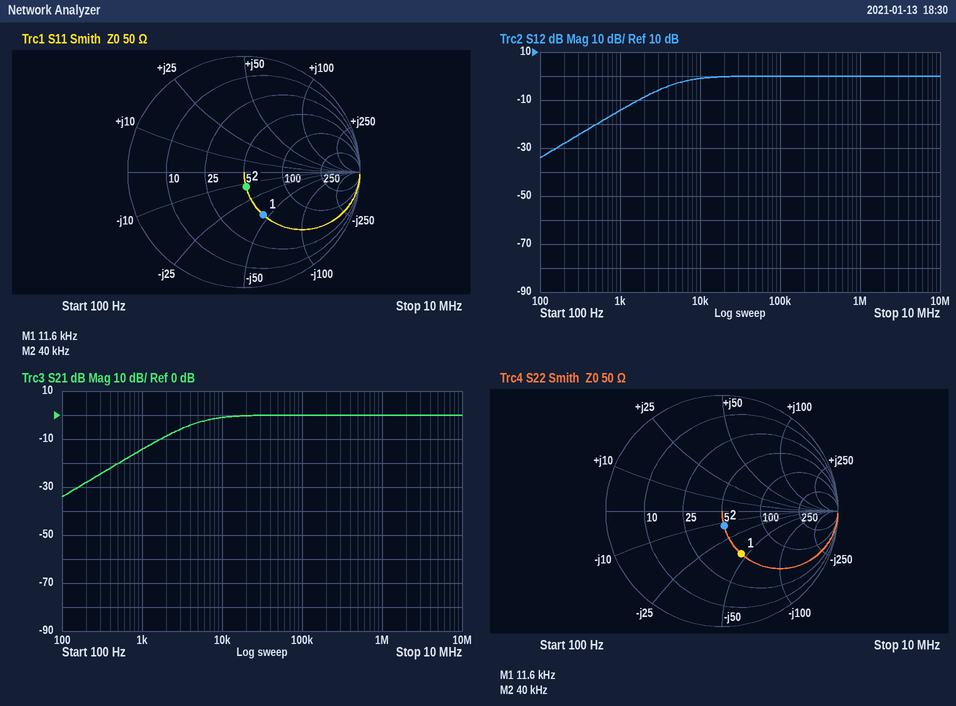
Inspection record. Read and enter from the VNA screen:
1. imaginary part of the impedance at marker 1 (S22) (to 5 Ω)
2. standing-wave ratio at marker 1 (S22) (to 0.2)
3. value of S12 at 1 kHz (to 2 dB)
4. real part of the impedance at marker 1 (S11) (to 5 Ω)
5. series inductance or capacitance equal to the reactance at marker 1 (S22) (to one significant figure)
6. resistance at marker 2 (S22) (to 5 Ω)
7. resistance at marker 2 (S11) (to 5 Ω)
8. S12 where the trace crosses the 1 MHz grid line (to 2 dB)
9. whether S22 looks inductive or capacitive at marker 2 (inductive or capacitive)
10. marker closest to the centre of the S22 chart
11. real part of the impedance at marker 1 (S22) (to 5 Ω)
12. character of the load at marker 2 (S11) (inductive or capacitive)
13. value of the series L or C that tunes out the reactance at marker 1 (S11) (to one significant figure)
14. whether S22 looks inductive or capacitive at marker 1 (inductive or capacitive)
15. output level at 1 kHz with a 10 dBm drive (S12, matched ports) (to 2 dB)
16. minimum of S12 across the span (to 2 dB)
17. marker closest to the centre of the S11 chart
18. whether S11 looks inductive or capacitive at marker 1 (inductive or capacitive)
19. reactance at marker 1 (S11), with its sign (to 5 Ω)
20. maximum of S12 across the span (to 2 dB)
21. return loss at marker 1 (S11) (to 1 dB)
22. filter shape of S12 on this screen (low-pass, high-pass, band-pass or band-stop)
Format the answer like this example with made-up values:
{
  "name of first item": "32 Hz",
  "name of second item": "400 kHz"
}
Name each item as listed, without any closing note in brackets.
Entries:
{
  "imaginary part of the impedance at marker 1 (S22)": "-45 Ω",
  "standing-wave ratio at marker 1 (S22)": "2.4",
  "value of S12 at 1 kHz": "-14 dB",
  "real part of the impedance at marker 1 (S11)": "50 Ω",
  "series inductance or capacitance equal to the reactance at marker 1 (S22)": "300 nF",
  "resistance at marker 2 (S22)": "50 Ω",
  "resistance at marker 2 (S11)": "50 Ω",
  "S12 where the trace crosses the 1 MHz grid line": "0 dB",
  "whether S22 looks inductive or capacitive at marker 2": "capacitive",
  "marker closest to the centre of the S22 chart": "marker 2",
  "real part of the impedance at marker 1 (S22)": "50 Ω",
  "character of the load at marker 2 (S11)": "capacitive",
  "value of the series L or C that tunes out the reactance at marker 1 (S11)": "600 µH",
  "whether S22 looks inductive or capacitive at marker 1": "capacitive",
  "output level at 1 kHz with a 10 dBm drive (S12, matched ports)": "-4 dBm",
  "minimum of S12 across the span": "-34 dB",
  "marker closest to the centre of the S11 chart": "marker 2",
  "whether S11 looks inductive or capacitive at marker 1": "capacitive",
  "reactance at marker 1 (S11), with its sign": "-45 Ω",
  "maximum of S12 across the span": "0 dB",
  "return loss at marker 1 (S11)": "8 dB",
  "filter shape of S12 on this screen": "high-pass"
}
